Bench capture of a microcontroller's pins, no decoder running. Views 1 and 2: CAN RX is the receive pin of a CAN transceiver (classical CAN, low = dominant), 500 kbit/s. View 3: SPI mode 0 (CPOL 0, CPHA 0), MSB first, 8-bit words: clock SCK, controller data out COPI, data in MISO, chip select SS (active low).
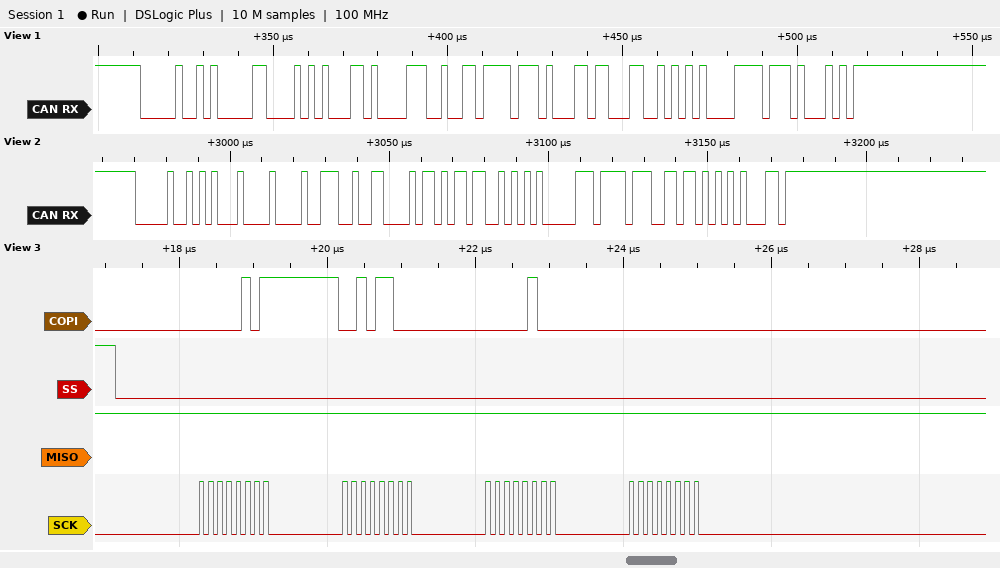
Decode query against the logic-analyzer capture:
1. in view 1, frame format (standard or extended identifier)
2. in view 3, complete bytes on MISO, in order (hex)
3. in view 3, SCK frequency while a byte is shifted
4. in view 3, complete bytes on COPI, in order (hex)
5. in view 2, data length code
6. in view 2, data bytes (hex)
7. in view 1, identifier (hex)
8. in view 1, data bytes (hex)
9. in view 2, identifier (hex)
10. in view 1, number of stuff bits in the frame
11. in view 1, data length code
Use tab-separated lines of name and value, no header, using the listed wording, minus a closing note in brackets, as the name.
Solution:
in view 1, frame format	standard
in view 3, complete bytes on MISO, in order	0xFF 0xFF 0xFF 0xFF
in view 3, SCK frequency while a byte is shifted	8 MHz
in view 3, complete bytes on COPI, in order	0x05 0x2C 0x04 0x00
in view 2, data length code	8
in view 2, data bytes	42 72 61 6B 65 50 6F 73
in view 1, identifier	0x014
in view 1, data bytes	54 68 72 6F 74 6C 65 50
in view 2, identifier	0x015
in view 1, number of stuff bits in the frame	2
in view 1, data length code	8
